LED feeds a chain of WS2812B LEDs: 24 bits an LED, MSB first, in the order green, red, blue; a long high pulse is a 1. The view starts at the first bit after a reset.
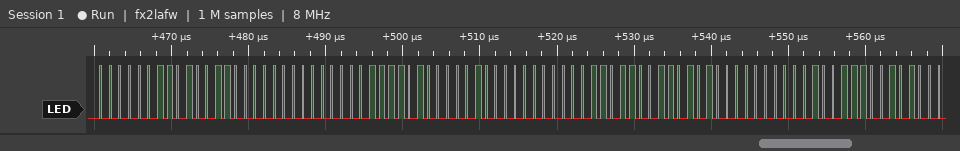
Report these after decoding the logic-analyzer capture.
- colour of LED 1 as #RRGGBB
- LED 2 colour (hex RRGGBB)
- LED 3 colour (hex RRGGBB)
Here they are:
#4C0300
#410F00
#351B00
